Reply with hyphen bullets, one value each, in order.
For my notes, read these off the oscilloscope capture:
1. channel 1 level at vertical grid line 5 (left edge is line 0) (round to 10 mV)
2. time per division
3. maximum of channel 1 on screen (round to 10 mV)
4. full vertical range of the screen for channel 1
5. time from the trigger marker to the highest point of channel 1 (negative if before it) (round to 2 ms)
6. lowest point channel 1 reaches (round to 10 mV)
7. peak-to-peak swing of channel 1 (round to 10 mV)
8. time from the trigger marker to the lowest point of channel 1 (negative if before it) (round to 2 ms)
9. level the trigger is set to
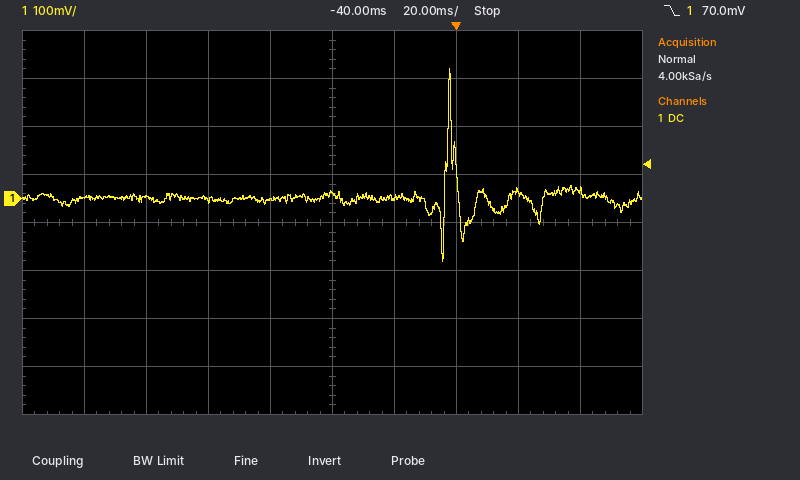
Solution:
- 10 mV
- 20 ms
- 270 mV
- 800 mV
- -2 ms
- -130 mV
- 400 mV
- -4 ms
- 70.0 mV
